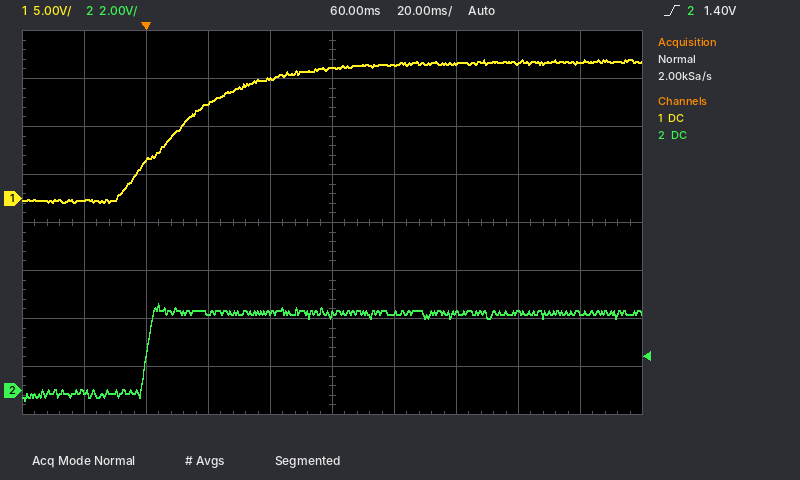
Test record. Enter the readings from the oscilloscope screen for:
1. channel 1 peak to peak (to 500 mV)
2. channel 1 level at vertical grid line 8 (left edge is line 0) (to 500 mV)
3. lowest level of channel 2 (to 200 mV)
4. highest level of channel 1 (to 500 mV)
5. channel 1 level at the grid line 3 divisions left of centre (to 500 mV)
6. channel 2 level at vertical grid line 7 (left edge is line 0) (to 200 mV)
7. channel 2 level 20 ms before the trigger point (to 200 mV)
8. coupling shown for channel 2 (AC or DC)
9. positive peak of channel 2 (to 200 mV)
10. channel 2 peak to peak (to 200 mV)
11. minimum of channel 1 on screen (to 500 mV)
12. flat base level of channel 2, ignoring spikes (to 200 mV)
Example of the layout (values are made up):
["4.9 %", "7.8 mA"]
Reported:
["15.0 V", "14.0 V", "-400 mV", "14.5 V", "4.0 V", "3.2 V", "0.0 V", "DC", "3.6 V", "4.0 V", "-500 mV", "-200 mV"]
